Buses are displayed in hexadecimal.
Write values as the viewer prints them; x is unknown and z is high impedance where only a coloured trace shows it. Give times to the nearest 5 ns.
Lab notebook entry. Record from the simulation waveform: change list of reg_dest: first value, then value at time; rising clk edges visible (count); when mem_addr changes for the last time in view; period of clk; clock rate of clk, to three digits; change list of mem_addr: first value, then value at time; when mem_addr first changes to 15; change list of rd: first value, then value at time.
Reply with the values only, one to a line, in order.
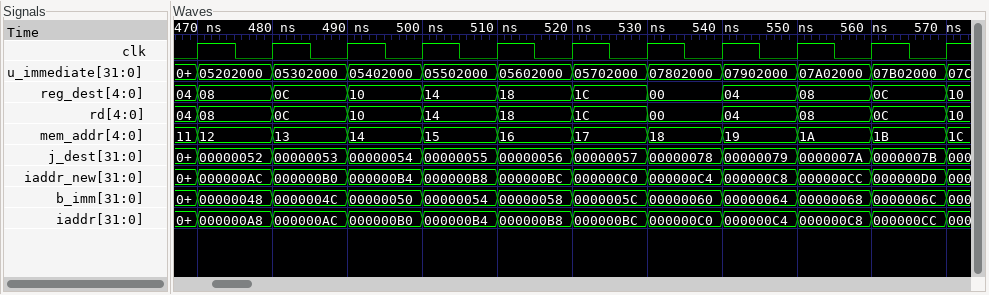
04, 08 at 470 ns, 0C at 480 ns, 10 at 490 ns, 14 at 500 ns, 18 at 510 ns, 1C at 520 ns, 00 at 530 ns, 04 at 540 ns, 08 at 550 ns, 0C at 560 ns, 10 at 570 ns
11
570 ns
10 ns
100 MHz
11, 12 at 470 ns, 13 at 480 ns, 14 at 490 ns, 15 at 500 ns, 16 at 510 ns, 17 at 520 ns, 18 at 530 ns, 19 at 540 ns, 1A at 550 ns, 1B at 560 ns, 1C at 570 ns
500 ns
04, 08 at 470 ns, 0C at 480 ns, 10 at 490 ns, 14 at 500 ns, 18 at 510 ns, 1C at 520 ns, 00 at 530 ns, 04 at 540 ns, 08 at 550 ns, 0C at 560 ns, 10 at 570 ns
